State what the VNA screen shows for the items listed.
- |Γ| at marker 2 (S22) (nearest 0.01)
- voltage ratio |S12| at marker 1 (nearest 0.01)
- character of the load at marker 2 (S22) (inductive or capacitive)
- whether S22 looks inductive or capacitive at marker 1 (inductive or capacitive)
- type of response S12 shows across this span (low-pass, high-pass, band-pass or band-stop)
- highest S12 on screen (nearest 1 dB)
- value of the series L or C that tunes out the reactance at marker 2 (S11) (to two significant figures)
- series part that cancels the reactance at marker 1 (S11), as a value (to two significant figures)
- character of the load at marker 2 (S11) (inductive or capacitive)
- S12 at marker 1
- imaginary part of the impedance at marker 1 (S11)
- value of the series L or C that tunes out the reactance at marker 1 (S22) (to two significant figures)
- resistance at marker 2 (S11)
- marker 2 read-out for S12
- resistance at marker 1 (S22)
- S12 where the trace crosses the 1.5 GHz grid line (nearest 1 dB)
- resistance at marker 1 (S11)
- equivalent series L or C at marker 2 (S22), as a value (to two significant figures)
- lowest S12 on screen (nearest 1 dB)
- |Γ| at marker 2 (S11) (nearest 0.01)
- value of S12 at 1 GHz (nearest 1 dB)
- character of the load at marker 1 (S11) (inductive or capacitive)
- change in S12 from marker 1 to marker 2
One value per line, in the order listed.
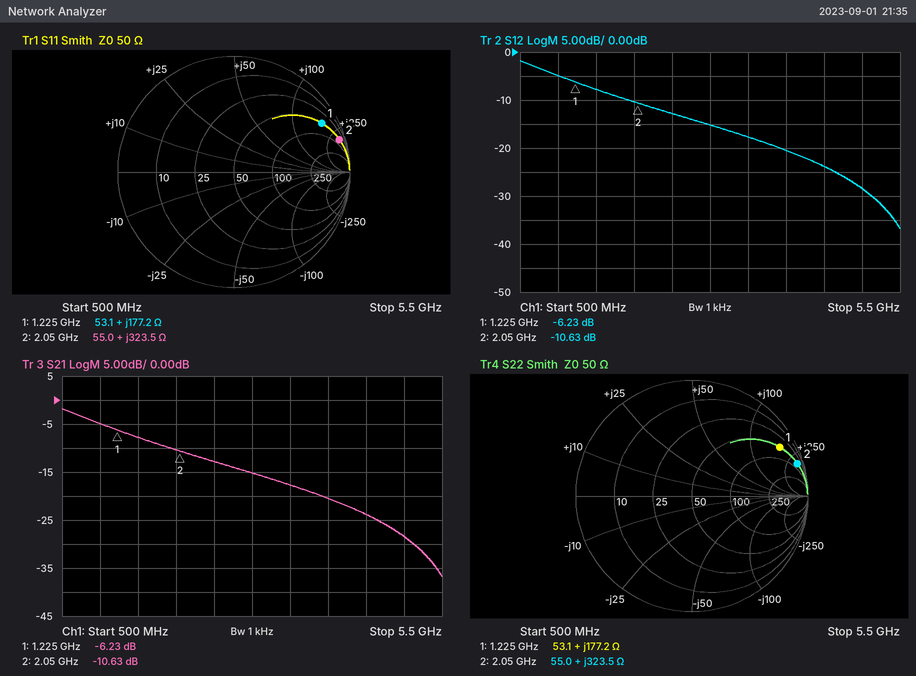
0.95
0.49
inductive
inductive
low-pass
-2 dB
240 fF
730 fF
inductive
-6.23 dB
+177.2 Ω
730 fF
55.0 Ω
-10.63 dB
53.1 Ω
-8 dB
53.1 Ω
25 nH
-37 dB
0.95
-5 dB
inductive
-4.40 dB
